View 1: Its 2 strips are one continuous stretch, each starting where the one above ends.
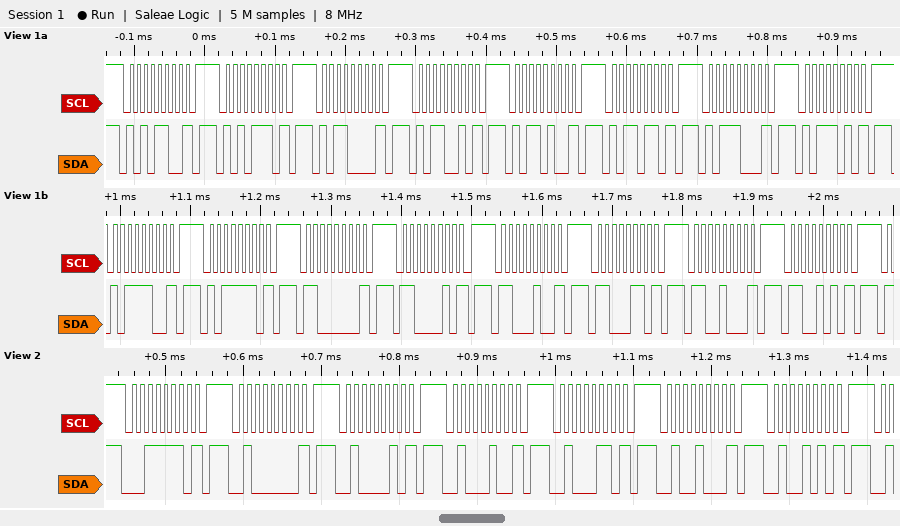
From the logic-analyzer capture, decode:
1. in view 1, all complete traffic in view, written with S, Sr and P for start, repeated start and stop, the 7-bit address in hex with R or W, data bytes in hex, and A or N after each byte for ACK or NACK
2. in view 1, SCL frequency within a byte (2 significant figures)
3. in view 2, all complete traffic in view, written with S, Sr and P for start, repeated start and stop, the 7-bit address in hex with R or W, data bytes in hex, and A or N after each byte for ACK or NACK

S 56W N P S 57W N P S 58W N P S 59W N P S 5AW N P S 5BW N P S 5CW N P S 5DW N P S 5EW N P S 5FW N P S 60W N P S 61W N P S 62W N P S 63W N P S 64W N P S 65W N P
100 kHz
S 1FW N P S 20W N P S 21W N P S 22W N P S 23W N P S 24W N P S 25W N P
